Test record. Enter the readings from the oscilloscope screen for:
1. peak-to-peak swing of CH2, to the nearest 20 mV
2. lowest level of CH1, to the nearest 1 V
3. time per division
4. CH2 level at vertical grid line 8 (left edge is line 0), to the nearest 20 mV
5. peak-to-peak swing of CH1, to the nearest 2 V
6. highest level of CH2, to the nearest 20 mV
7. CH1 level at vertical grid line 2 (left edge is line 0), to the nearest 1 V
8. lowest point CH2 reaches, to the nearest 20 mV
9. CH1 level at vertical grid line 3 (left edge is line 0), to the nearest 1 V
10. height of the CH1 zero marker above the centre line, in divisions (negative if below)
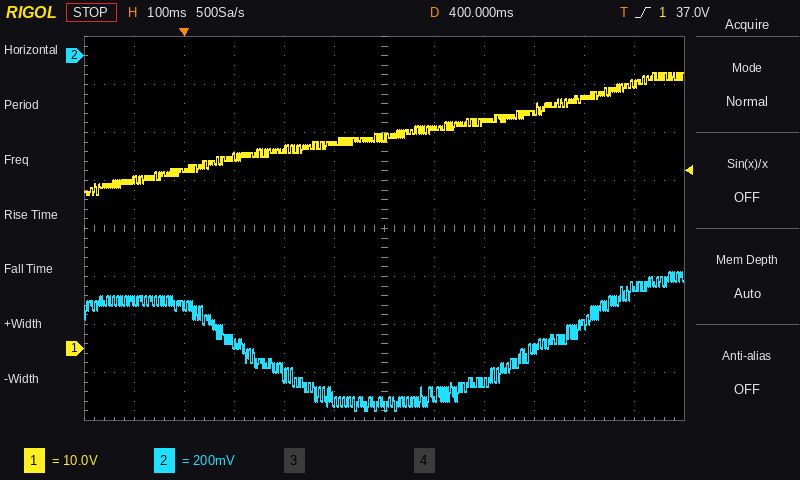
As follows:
580 mV
32 V
100 ms
-1.36 V
26 V
-900 mV
37 V
-1.48 V
40 V
-2.5 div
